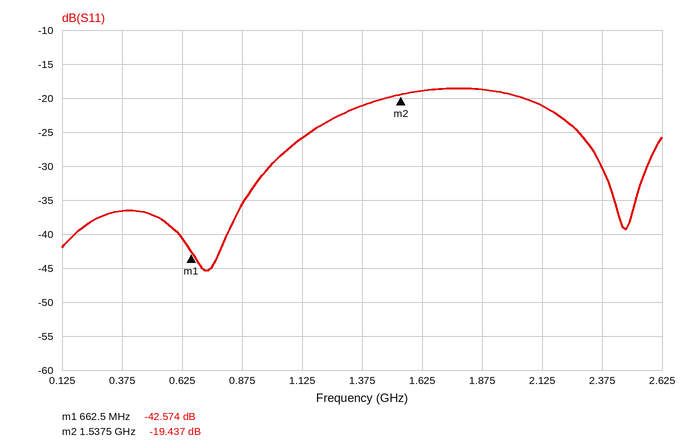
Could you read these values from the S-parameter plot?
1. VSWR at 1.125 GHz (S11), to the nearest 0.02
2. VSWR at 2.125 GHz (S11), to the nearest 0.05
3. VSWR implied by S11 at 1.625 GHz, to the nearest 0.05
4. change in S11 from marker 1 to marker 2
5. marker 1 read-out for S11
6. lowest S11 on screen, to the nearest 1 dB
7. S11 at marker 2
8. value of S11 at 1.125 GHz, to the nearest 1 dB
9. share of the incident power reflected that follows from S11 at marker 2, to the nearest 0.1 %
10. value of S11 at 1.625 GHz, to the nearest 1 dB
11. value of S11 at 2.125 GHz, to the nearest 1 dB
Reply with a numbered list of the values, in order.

1. 1.10
2. 1.20
3. 1.25
4. 23.137 dB
5. -42.574 dB
6. -45 dB
7. -19.437 dB
8. -26 dB
9. 1.1 %
10. -19 dB
11. -21 dB
